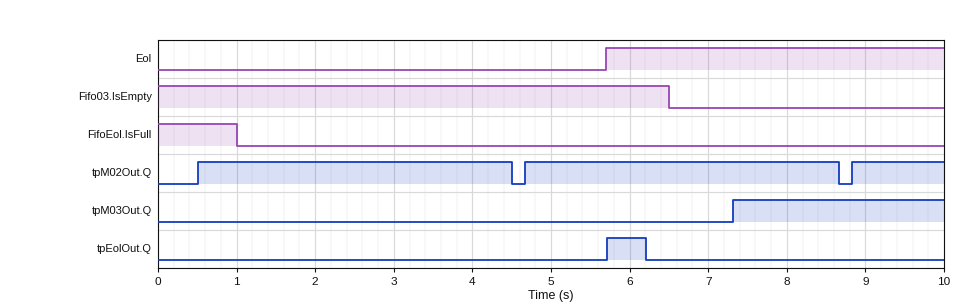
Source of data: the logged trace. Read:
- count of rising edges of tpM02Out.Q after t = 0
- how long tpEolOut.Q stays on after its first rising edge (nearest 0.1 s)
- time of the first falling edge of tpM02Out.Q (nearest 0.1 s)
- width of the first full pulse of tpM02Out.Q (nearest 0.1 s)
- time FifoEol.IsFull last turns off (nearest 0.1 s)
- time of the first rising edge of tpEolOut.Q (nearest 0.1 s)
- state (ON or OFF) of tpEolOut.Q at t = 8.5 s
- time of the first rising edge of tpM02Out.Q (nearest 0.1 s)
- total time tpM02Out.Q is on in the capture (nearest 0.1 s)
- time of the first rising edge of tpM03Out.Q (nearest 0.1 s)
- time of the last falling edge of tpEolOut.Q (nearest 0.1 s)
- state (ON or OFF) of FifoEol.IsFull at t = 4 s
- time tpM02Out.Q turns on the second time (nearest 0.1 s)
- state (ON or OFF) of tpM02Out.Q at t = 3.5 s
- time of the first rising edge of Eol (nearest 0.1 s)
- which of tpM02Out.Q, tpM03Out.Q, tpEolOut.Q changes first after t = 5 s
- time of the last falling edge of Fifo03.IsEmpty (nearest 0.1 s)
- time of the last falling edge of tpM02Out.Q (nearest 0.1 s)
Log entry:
3
0.5 s
4.5 s
4.0 s
1.0 s
5.7 s
OFF
0.5 s
9.2 s
7.3 s
6.2 s
OFF
4.7 s
ON
5.7 s
tpEolOut.Q
6.5 s
8.7 s
